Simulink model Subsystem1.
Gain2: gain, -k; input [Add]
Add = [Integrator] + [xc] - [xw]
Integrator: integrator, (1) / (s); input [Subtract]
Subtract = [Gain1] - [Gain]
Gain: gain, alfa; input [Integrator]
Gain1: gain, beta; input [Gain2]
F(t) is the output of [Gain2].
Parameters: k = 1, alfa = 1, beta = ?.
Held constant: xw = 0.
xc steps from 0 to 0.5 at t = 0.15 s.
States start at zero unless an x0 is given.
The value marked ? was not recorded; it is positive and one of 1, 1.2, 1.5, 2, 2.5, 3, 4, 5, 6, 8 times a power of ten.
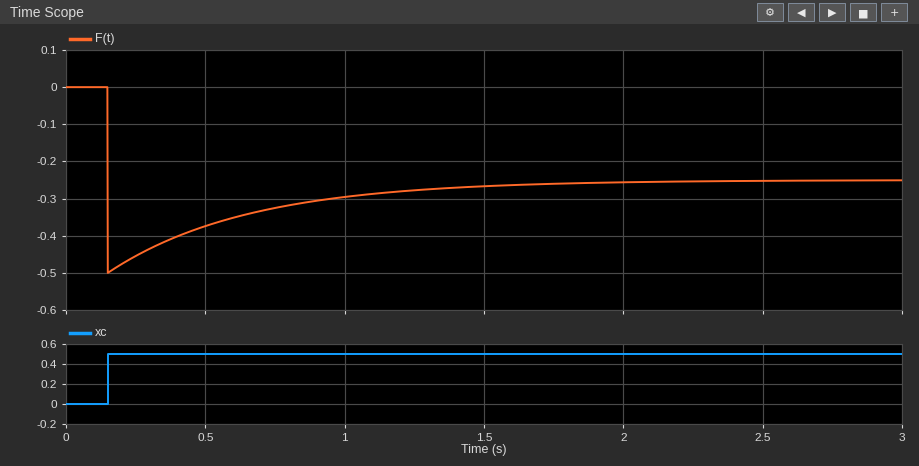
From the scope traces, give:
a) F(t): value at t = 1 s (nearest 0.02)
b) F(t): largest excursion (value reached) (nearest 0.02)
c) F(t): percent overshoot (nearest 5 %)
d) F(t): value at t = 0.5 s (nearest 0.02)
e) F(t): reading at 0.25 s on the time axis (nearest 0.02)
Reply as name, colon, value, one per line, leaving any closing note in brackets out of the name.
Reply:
F(t): value at t = 1 s: -0.30
F(t): largest excursion (value reached): -0.50
F(t): percent overshoot: 100 %
F(t): value at t = 0.5 s: -0.38
F(t): reading at 0.25 s on the time axis: -0.46
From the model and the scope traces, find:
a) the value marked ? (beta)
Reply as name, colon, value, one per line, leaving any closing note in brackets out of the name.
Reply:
the value marked ?: 1
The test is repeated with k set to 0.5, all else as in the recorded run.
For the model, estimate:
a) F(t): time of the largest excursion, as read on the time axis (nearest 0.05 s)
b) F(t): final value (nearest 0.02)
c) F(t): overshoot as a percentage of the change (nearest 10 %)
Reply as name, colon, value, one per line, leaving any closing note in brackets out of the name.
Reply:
F(t): time of the largest excursion, as read on the time axis: 0.15 s
F(t): final value: -0.16
F(t): overshoot as a percentage of the change: 50 %
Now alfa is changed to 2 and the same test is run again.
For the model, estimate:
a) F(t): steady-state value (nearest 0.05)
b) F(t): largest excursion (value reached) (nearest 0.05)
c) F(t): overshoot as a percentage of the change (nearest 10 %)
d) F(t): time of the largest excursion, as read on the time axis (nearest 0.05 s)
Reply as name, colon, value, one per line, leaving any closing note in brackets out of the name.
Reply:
F(t): steady-state value: -0.35
F(t): largest excursion (value reached): -0.50
F(t): overshoot as a percentage of the change: 50 %
F(t): time of the largest excursion, as read on the time axis: 0.15 s
